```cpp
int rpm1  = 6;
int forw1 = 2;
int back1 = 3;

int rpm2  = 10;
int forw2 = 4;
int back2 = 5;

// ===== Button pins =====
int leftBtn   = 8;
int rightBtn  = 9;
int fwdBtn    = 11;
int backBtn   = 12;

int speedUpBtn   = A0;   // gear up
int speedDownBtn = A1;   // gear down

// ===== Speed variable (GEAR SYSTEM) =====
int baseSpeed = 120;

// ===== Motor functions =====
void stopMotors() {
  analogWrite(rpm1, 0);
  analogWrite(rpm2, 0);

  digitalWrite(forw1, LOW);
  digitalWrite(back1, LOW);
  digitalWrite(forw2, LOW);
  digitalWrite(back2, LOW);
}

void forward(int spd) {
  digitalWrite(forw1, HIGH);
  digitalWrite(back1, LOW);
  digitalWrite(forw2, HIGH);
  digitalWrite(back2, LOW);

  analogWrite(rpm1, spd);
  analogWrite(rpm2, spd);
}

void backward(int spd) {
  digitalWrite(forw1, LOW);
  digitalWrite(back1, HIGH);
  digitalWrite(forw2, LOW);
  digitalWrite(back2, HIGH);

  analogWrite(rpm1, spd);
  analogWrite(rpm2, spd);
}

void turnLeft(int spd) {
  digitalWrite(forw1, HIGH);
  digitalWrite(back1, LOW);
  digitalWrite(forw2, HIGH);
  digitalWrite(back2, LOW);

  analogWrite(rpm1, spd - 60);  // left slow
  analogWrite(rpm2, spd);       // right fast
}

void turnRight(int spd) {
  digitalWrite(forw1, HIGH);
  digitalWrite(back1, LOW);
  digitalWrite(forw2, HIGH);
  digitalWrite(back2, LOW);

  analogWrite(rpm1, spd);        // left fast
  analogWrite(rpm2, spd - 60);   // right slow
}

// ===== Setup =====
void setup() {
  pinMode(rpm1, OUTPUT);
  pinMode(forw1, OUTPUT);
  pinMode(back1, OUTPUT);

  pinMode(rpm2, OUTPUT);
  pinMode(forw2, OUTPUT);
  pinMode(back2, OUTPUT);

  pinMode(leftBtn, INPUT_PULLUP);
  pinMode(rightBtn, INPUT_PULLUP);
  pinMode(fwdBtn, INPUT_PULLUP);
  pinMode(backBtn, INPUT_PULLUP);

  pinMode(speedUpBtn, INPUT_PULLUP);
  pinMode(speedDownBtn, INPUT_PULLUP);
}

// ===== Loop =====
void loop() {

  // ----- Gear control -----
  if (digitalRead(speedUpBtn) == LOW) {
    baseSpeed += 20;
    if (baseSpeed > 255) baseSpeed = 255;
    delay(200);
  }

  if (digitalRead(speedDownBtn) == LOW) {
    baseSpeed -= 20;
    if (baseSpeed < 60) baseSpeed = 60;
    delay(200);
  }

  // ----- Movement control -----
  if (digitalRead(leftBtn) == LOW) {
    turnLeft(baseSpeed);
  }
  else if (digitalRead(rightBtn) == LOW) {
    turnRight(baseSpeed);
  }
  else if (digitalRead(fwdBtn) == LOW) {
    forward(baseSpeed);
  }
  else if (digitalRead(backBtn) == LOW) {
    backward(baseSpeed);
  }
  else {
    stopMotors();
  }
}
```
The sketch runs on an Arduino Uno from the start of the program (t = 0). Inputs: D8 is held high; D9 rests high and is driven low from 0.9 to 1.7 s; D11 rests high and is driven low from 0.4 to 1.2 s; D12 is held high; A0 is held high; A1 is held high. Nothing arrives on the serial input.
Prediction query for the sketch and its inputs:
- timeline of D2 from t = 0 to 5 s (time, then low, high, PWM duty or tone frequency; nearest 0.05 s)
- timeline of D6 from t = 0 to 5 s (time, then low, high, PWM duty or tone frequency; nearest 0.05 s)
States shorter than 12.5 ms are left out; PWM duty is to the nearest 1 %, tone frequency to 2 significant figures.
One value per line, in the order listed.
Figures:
0 s low; 0.4 s high; 1.7 s low
0 s low; 0.4 s PWM 47 %; 1.7 s low
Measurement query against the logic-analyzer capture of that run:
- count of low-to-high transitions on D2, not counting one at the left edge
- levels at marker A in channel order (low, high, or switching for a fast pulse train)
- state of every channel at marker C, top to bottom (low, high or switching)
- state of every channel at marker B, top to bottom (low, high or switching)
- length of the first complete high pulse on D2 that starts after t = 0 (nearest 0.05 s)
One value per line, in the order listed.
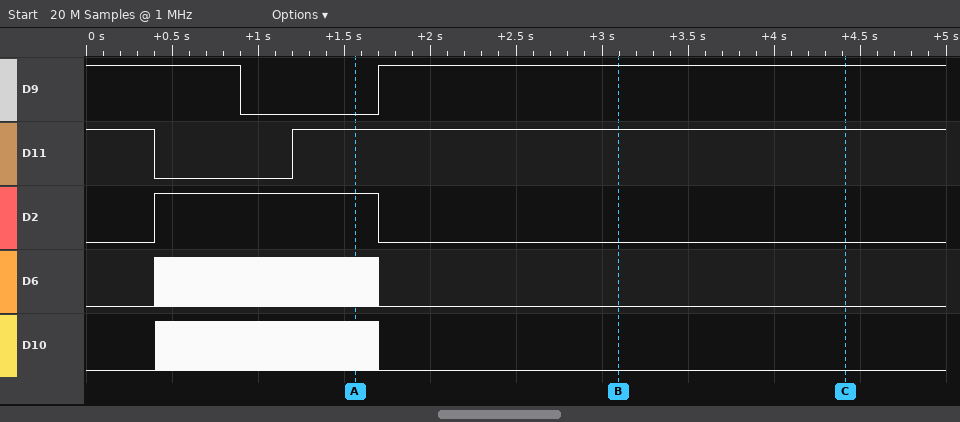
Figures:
1
D9 low, D11 high, D2 high, D6 switching, D10 switching
D9 high, D11 high, D2 low, D6 low, D10 low
D9 high, D11 high, D2 low, D6 low, D10 low
1.30 s
